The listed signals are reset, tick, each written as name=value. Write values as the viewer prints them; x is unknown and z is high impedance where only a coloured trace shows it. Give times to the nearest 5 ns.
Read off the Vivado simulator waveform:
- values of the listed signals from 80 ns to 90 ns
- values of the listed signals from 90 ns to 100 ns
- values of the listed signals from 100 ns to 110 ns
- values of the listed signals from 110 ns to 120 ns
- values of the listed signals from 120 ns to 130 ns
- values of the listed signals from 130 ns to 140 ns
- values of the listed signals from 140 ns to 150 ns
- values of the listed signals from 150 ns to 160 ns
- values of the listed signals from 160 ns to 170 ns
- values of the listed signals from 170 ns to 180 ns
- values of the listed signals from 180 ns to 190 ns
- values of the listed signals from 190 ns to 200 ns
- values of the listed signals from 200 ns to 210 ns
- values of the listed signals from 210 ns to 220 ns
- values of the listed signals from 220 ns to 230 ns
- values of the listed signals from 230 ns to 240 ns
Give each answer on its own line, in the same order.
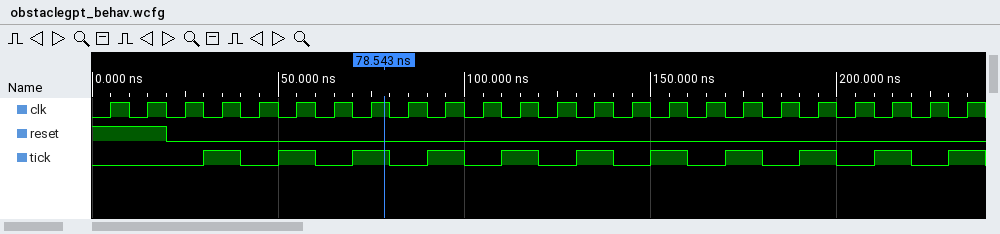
reset=0, tick=0
reset=0, tick=1
reset=0, tick=0
reset=0, tick=1
reset=0, tick=0
reset=0, tick=1
reset=0, tick=0
reset=0, tick=1
reset=0, tick=0
reset=0, tick=1
reset=0, tick=0
reset=0, tick=1
reset=0, tick=0
reset=0, tick=1
reset=0, tick=0
reset=0, tick=1
